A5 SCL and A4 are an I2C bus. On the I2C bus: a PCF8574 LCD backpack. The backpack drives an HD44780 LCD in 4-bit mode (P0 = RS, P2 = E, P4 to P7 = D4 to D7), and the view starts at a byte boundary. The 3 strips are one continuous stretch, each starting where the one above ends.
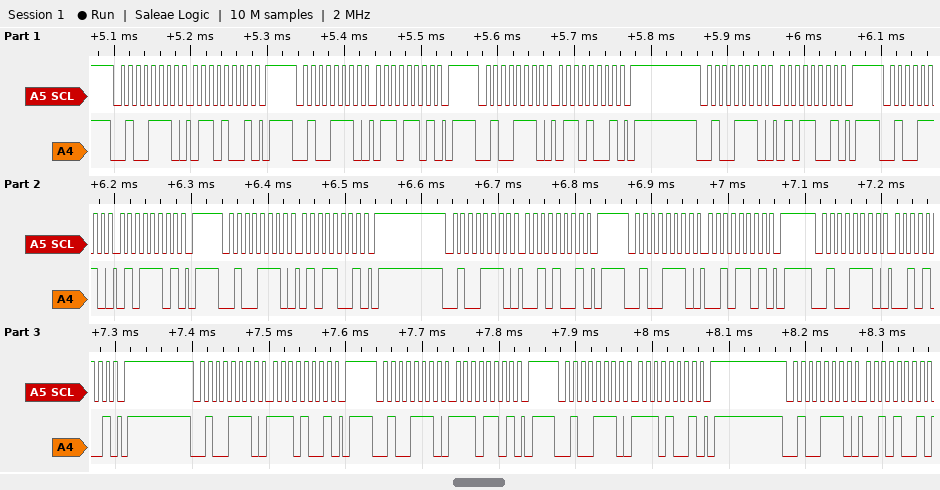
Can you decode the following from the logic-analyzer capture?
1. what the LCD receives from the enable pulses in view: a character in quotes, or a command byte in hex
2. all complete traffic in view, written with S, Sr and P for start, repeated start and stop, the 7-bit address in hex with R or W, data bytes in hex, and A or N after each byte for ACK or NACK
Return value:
'e' '.'
S 27W A 69 A P S 27W A 6D A P S 27W A 69 A P S 27W A 59 A P S 27W A 5D A P S 27W A 59 A P S 27W A 29 A P S 27W A 2D A P S 27W A 29 A P S 27W A E9 A P S 27W A ED A P S 27W A E9 A P S 27W A 29 A
